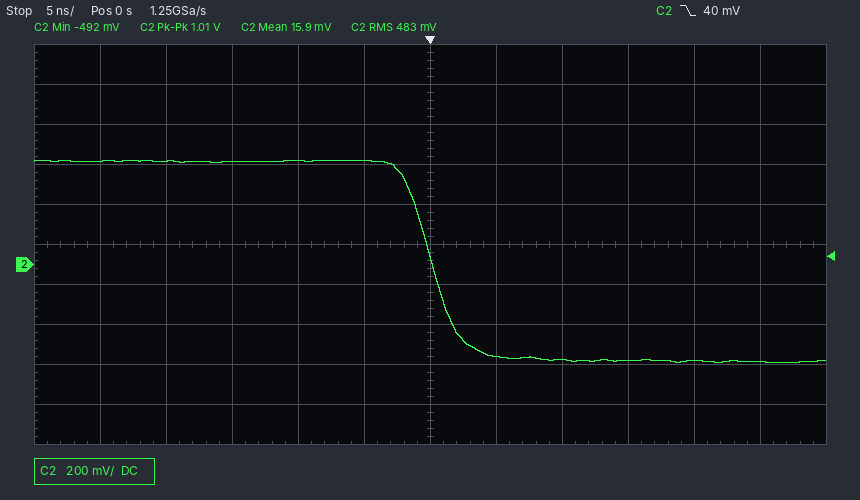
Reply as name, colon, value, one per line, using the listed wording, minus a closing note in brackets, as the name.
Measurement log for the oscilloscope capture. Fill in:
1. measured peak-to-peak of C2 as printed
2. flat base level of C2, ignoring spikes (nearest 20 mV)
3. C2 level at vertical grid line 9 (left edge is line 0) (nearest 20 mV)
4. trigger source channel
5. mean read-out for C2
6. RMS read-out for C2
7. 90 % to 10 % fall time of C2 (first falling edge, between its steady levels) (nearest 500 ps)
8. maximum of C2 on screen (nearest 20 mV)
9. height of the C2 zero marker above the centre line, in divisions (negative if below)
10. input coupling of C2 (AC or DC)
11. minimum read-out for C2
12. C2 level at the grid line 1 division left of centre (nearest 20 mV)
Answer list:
measured peak-to-peak of C2 as printed: 1.01 V
flat base level of C2, ignoring spikes: -480 mV
C2 level at vertical grid line 9 (left edge is line 0): -480 mV
trigger source channel: C2
mean read-out for C2: 15.9 mV
RMS read-out for C2: 483 mV
90 % to 10 % fall time of C2 (first falling edge, between its steady levels): 4.5 ns
maximum of C2 on screen: 520 mV
height of the C2 zero marker above the centre line, in divisions: -0.5 div
input coupling of C2: DC
minimum read-out for C2: -492 mV
C2 level at the grid line 1 division left of centre: 520 mV
